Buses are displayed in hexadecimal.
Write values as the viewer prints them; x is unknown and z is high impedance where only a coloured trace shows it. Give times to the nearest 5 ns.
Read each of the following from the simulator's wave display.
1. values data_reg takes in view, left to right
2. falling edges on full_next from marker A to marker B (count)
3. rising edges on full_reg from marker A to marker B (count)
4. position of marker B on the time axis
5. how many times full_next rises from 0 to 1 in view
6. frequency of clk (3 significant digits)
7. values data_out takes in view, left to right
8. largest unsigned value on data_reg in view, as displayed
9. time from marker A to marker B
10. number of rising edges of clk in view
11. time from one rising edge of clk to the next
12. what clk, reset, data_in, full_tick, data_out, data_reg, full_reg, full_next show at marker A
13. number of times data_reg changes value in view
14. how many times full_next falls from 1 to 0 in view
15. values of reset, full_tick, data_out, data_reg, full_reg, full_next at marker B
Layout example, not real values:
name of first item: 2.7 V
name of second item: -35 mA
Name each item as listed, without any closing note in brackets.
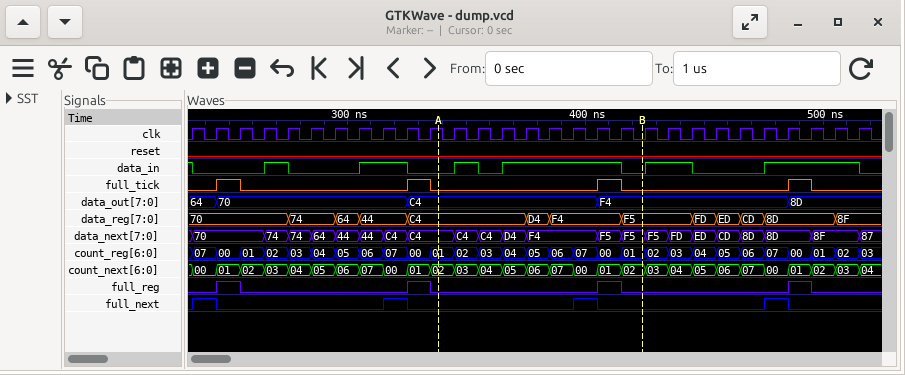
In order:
values data_reg takes in view, left to right: 70, 74, 64, 44, C4, D4, F4, F5, FD, ED, CD, 8D, 8F
falling edges on full_next from marker A to marker B: 1
rising edges on full_reg from marker A to marker B: 1
position of marker B on the time axis: 425 ns
how many times full_next rises from 0 to 1 in view: 4
frequency of clk: 100 MHz
values data_out takes in view, left to right: 64, 70, C4, F4, 8D
largest unsigned value on data_reg in view, as displayed: FD
time from marker A to marker B: 85 ns
number of rising edges of clk in view: 29
time from one rising edge of clk to the next: 10 ns
what clk, reset, data_in, full_tick, data_out, data_reg, full_reg, full_next show at marker A: clk=1, reset=0, data_in=0, full_tick=0, data_out=C4, data_reg=C4, full_reg=0, full_next=0
number of times data_reg changes value in view: 12
how many times full_next falls from 1 to 0 in view: 4
values of reset, full_tick, data_out, data_reg, full_reg, full_next at marker B: reset=0, full_tick=0, data_out=F4, data_reg=F5, full_reg=0, full_next=0
